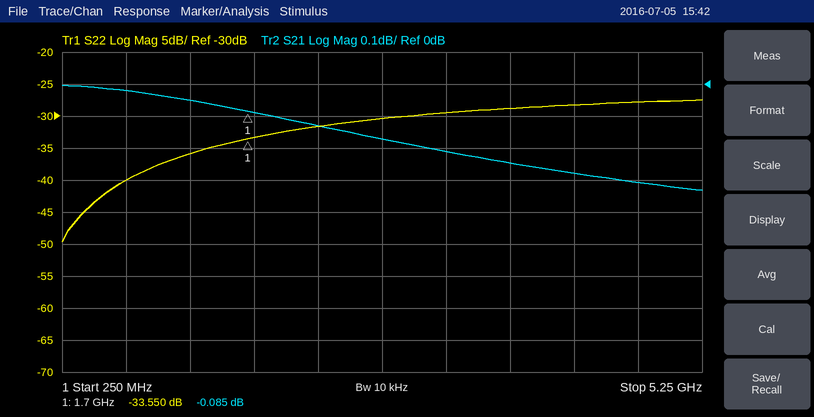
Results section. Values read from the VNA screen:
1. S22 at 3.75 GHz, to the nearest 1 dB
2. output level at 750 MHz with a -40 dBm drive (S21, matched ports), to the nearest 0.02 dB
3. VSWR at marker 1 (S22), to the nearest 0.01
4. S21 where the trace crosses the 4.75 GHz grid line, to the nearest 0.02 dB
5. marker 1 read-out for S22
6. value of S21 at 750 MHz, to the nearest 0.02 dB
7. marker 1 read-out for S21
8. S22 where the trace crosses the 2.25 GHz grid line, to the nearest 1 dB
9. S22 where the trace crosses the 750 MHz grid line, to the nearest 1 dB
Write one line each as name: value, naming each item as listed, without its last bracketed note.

S22 at 3.75 GHz, to the nearest 1 dB: -29 dB
output level at 750 MHz with a -40 dBm drive (S21, matched ports), to the nearest 0.02 dB: -40.02 dBm
VSWR at marker 1 (S22), to the nearest 0.01: 1.04
S21 where the trace crosses the 4.75 GHz grid line, to the nearest 0.02 dB: -0.30 dB
marker 1 read-out for S22: -33.550 dB
value of S21 at 750 MHz, to the nearest 0.02 dB: -0.02 dB
marker 1 read-out for S21: -0.085 dB
S22 where the trace crosses the 2.25 GHz grid line, to the nearest 1 dB: -32 dB
S22 where the trace crosses the 750 MHz grid line, to the nearest 1 dB: -40 dB
